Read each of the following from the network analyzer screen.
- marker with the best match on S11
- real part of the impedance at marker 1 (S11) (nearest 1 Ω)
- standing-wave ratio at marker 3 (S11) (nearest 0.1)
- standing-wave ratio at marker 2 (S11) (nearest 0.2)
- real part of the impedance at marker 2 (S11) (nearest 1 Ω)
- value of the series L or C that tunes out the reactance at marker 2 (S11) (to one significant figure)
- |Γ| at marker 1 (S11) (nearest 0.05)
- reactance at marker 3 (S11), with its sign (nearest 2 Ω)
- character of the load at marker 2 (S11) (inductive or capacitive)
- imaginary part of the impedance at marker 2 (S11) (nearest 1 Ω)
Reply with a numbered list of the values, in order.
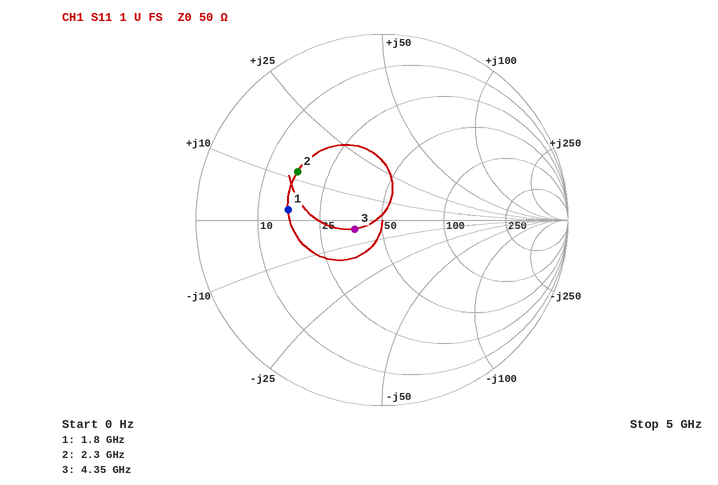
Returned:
1. marker 3
2. 16 Ω
3. 1.4
4. 3.2
5. 17 Ω
6. 6 pF
7. 0.50
8. -4 Ω
9. inductive
10. +12 Ω
